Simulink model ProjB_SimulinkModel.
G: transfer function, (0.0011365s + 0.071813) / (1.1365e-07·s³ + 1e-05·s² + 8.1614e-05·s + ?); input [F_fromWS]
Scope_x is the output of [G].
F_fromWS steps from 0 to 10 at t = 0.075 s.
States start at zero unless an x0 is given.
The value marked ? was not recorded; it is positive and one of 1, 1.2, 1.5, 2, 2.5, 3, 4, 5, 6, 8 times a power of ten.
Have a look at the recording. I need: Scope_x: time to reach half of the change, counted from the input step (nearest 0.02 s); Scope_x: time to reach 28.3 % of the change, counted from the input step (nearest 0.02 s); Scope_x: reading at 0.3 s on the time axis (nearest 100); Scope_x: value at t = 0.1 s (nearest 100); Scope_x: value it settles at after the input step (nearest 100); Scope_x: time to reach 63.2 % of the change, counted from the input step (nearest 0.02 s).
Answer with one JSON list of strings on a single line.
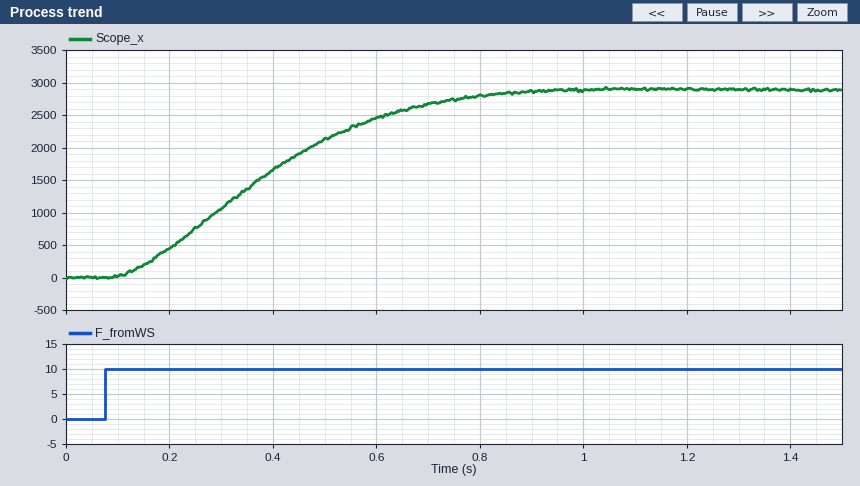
["0.28 s", "0.18 s", "1100", "0", "2900", "0.36 s"]
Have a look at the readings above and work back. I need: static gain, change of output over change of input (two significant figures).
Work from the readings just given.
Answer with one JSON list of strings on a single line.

["290"]
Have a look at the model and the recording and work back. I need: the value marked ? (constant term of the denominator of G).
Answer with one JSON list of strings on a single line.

["0.00025"]
